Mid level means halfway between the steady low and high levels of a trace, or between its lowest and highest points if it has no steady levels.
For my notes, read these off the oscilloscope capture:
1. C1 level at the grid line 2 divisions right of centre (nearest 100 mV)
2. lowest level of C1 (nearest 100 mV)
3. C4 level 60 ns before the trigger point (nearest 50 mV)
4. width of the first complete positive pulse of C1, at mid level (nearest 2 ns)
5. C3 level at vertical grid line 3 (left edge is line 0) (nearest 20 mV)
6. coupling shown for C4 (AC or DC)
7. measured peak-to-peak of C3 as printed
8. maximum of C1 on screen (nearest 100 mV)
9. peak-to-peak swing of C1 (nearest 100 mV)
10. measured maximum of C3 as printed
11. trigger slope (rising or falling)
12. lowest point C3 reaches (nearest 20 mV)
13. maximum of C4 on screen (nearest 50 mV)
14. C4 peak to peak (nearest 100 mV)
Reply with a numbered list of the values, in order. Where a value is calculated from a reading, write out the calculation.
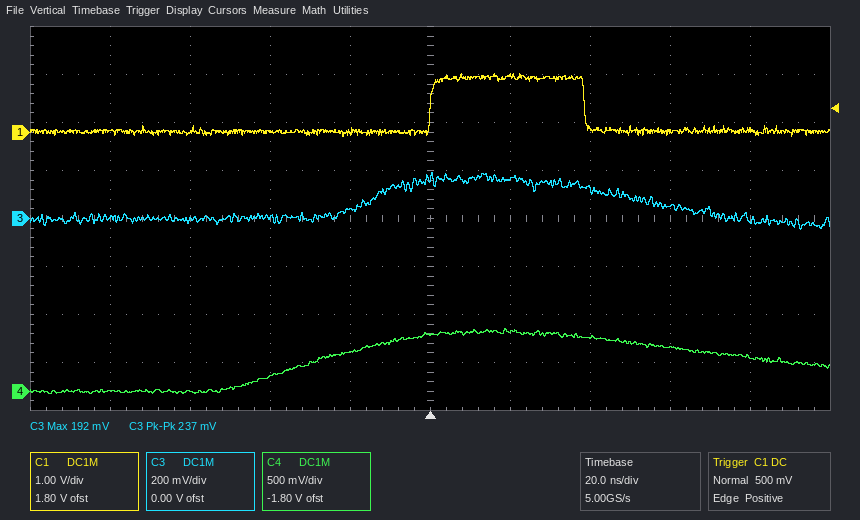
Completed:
1. 100 mV
2. -100 mV
3. 0 mV
4. 38 ns
5. 0 mV
6. DC
7. 237 mV
8. 1.2 V
9. 1.2 V − (-100 mV) = 1.3 V
10. 192 mV
11. rising
12. -40 mV
13. 650 mV
14. 700 mV
